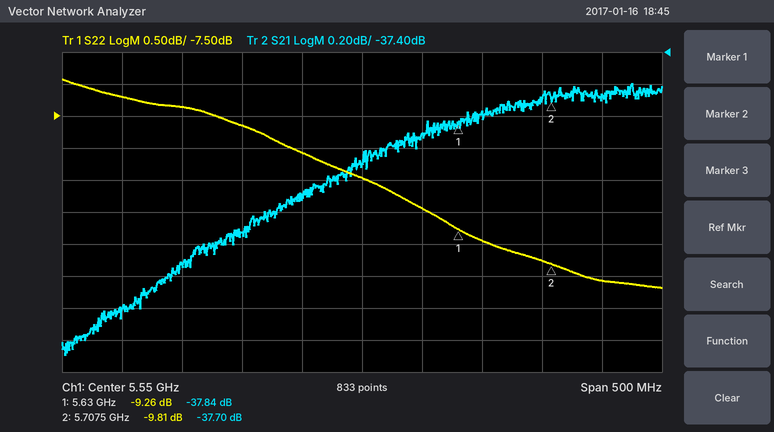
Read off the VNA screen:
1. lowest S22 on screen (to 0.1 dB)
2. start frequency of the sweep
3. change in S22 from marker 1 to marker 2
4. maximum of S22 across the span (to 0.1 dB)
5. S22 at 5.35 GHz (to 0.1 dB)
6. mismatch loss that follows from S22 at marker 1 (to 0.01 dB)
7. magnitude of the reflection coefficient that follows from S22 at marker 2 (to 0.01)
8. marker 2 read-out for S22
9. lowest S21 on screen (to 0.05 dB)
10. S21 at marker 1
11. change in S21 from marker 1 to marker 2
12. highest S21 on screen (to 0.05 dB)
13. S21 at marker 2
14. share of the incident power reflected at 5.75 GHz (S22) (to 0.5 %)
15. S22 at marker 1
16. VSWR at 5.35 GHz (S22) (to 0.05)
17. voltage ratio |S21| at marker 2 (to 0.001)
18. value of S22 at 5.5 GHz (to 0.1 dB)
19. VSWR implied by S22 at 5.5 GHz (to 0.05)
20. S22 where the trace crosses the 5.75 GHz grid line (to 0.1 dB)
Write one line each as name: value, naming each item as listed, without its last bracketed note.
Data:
lowest S22 on screen: -10.2 dB
start frequency of the sweep: 5.3 GHz
change in S22 from marker 1 to marker 2: -0.55 dB
maximum of S22 across the span: -6.9 dB
S22 at 5.35 GHz: -7.2 dB
mismatch loss that follows from S22 at marker 1: 0.55 dB
magnitude of the reflection coefficient that follows from S22 at marker 2: 0.32
marker 2 read-out for S22: -9.81 dB
lowest S21 on screen: -39.30 dB
S21 at marker 1: -37.84 dB
change in S21 from marker 1 to marker 2: 0.14 dB
highest S21 on screen: -37.60 dB
S21 at marker 2: -37.70 dB
share of the incident power reflected at 5.75 GHz (S22): 10.0 %
S22 at marker 1: -9.26 dB
VSWR at 5.35 GHz (S22): 2.55
voltage ratio |S21| at marker 2: 0.013
value of S22 at 5.5 GHz: -8.1 dB
VSWR implied by S22 at 5.5 GHz: 2.30
S22 where the trace crosses the 5.75 GHz grid line: -10.1 dB
